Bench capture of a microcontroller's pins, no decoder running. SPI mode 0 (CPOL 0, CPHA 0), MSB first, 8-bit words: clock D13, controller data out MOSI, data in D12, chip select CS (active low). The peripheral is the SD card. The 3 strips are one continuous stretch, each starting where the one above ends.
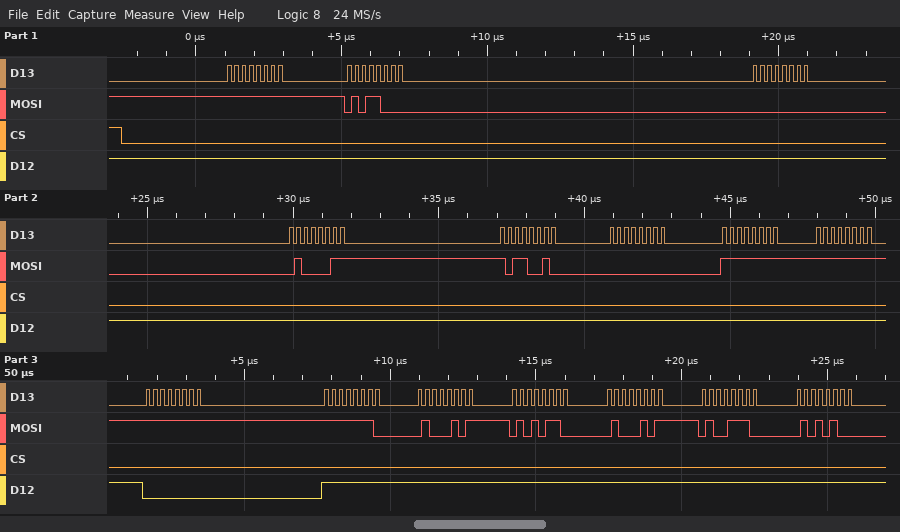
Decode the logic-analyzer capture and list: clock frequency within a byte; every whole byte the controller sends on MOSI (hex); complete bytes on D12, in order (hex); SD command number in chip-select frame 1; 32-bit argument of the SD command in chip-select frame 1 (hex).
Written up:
4 MHz
FF 58 00 43 B2 00 FF FF FF FE 45 56 45 4E 54
FF FF FF FF FF FF FF FF 00 FF FF FF FF FF FF
CMD24
0x0043B200
